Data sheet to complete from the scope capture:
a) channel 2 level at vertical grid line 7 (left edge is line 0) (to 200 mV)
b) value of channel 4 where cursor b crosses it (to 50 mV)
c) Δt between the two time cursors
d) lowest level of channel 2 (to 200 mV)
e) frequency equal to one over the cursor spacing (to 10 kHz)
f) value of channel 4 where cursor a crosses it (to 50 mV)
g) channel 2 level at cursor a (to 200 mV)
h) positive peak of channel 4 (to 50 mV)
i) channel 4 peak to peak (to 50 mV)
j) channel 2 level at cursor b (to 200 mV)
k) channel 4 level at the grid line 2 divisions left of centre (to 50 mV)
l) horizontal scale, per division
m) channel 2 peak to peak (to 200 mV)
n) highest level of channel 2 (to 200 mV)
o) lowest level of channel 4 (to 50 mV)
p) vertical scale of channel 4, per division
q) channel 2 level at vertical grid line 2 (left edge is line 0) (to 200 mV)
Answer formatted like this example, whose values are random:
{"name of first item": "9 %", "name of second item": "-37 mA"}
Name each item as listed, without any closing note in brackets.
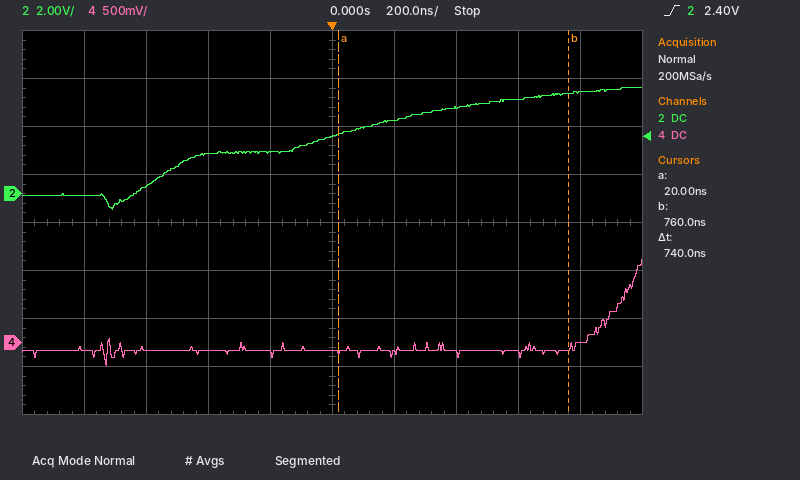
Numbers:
{"channel 2 level at vertical grid line 7 (left edge is line 0)": "3.6 V", "value of channel 4 where cursor b crosses it": "-50 mV", "Δt between the two time cursors": "740 ns", "lowest level of channel 2": "-600 mV", "frequency equal to one over the cursor spacing": "1.35 MHz", "value of channel 4 where cursor a crosses it": "-100 mV", "channel 2 level at cursor a": "2.4 V", "positive peak of channel 4": "850 mV", "channel 4 peak to peak": "1.10 V", "channel 2 level at cursor b": "4.2 V", "channel 4 level at the grid line 2 divisions left of centre": "-100 mV", "horizontal scale, per division": "200 ns", "channel 2 peak to peak": "5.0 V", "highest level of channel 2": "4.4 V", "lowest level of channel 4": "-250 mV", "vertical scale of channel 4, per division": "500 mV", "channel 2 level at vertical grid line 2 (left edge is line 0)": "400 mV"}
